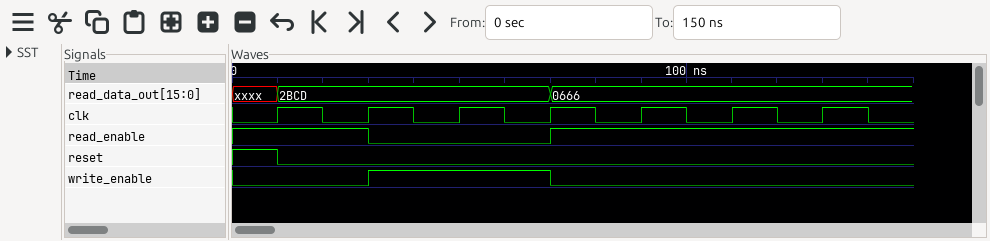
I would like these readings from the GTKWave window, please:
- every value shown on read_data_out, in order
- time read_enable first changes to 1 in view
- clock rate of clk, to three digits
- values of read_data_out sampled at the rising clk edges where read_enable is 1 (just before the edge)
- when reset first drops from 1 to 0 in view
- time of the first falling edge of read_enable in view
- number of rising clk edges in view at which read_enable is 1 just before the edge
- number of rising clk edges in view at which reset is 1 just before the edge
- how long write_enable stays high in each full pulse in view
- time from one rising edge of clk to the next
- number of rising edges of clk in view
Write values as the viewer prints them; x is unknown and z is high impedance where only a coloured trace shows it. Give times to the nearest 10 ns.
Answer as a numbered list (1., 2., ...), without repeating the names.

1. xxxx, 2BCD, 0666
2. 70 ns
3. 50.0 MHz
4. xxxx, 2BCD, 0666, 0666, 0666
5. 10 ns
6. 30 ns
7. 5
8. 1
9. 40 ns
10. 20 ns
11. 7
